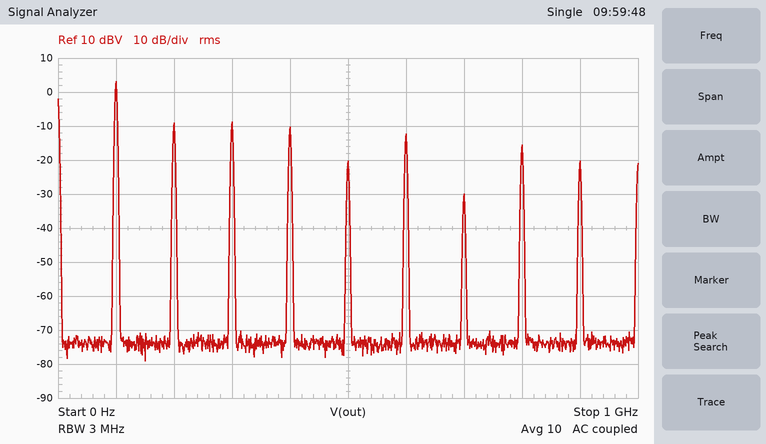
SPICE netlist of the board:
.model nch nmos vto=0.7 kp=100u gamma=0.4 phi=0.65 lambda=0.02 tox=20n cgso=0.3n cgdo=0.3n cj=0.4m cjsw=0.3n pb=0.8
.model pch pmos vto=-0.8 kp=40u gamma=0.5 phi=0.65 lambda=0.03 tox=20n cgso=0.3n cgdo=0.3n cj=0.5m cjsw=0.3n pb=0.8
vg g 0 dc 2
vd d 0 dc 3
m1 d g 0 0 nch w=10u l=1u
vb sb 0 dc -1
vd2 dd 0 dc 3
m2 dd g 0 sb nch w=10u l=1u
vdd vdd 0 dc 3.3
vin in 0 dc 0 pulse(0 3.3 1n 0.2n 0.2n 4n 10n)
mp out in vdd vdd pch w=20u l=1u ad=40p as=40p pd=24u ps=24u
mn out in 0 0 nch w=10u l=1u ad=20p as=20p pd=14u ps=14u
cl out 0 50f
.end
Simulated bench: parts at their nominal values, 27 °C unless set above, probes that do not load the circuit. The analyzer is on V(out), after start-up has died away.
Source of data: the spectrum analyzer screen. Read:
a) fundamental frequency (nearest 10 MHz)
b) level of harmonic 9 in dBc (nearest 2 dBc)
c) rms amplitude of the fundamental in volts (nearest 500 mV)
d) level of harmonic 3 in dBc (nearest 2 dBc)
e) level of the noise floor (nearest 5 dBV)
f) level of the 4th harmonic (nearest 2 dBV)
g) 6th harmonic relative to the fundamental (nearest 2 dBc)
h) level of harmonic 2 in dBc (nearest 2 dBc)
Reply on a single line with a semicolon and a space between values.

100 MHz; -24 dBc; 1.5 V; -12 dBc; -75 dBV; -10 dBV; -16 dBc; -12 dBc
